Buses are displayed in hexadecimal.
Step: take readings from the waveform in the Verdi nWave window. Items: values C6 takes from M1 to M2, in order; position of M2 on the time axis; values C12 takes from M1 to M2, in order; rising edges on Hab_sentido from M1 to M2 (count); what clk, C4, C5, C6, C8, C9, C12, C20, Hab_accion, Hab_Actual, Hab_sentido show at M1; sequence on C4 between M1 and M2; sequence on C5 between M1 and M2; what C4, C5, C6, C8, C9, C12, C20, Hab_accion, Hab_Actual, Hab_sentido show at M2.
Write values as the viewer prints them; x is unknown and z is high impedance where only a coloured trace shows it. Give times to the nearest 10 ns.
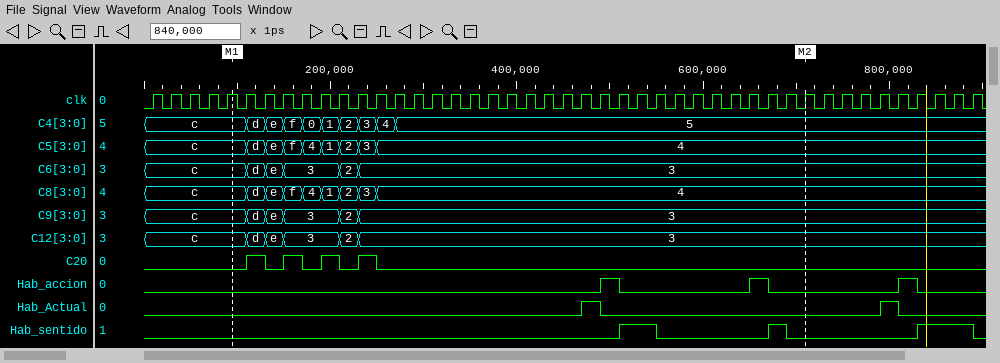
c, d, e, 3, 2, 3
710 ns
c, d, e, 3, 2, 3
2
clk=1, C4=c, C5=c, C6=c, C8=c, C9=c, C12=c, C20=0, Hab_accion=0, Hab_Actual=0, Hab_sentido=0
c, d, e, f, 0, 1, 2, 3, 4, 5
c, d, e, f, 4, 1, 2, 3, 4
C4=5, C5=4, C6=3, C8=4, C9=3, C12=3, C20=0, Hab_accion=0, Hab_Actual=0, Hab_sentido=0
